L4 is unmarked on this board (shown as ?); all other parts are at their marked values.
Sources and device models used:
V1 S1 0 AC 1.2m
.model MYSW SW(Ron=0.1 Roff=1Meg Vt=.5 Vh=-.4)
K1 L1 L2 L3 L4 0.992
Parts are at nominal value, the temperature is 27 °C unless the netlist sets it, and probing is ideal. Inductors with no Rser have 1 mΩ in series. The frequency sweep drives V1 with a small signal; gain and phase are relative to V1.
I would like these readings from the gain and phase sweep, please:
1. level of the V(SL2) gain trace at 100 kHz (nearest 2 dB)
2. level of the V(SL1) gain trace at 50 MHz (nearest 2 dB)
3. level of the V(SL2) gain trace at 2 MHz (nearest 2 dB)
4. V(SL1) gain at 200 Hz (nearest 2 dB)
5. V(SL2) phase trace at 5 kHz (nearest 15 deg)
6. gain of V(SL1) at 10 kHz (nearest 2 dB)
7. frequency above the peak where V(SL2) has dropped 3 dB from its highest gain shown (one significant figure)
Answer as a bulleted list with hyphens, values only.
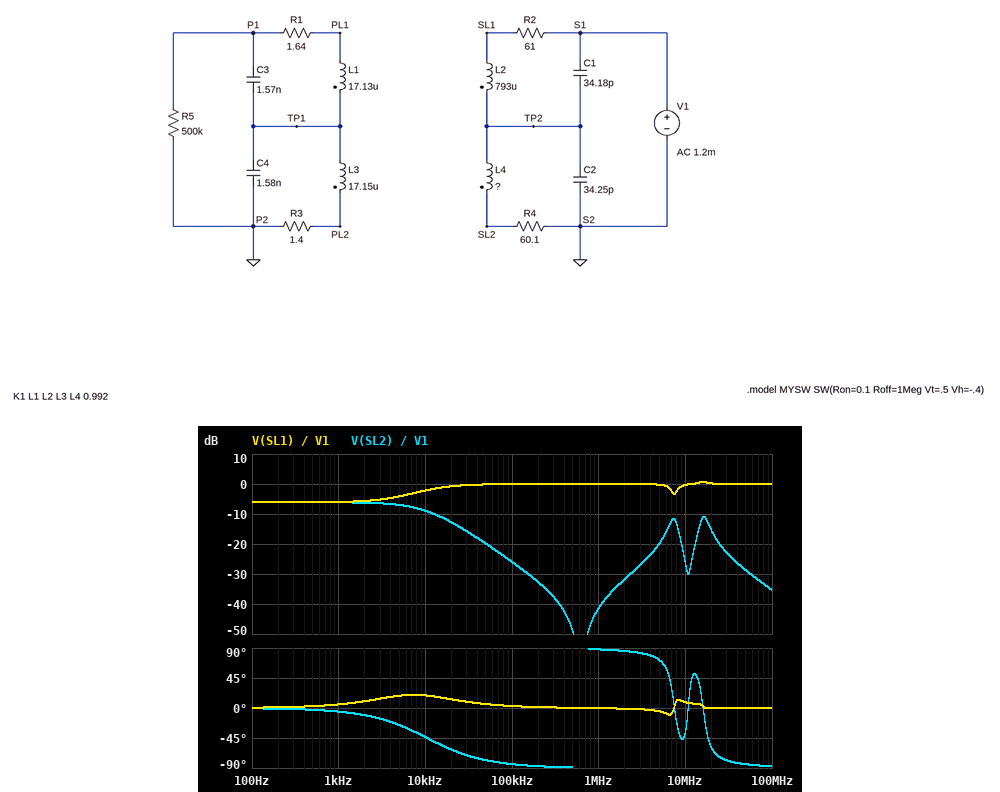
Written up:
- -26 dB
- 0 dB
- -32 dB
- -6 dB
- -30 deg
- -2 dB
- 10 kHz
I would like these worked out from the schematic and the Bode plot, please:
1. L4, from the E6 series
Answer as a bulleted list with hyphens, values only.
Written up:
- 220 µH
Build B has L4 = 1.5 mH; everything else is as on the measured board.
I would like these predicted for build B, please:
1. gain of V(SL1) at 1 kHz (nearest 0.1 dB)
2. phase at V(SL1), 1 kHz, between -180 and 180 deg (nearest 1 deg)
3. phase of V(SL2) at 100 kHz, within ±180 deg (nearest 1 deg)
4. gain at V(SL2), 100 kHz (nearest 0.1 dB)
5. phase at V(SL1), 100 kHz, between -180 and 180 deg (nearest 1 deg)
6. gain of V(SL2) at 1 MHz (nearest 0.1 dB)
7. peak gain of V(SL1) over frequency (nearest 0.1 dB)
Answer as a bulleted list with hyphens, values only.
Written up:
- -5.5 dB
- 12 deg
- -88 deg
- -33.5 dB
- 1 deg
- -56.0 dB
- 0 dB
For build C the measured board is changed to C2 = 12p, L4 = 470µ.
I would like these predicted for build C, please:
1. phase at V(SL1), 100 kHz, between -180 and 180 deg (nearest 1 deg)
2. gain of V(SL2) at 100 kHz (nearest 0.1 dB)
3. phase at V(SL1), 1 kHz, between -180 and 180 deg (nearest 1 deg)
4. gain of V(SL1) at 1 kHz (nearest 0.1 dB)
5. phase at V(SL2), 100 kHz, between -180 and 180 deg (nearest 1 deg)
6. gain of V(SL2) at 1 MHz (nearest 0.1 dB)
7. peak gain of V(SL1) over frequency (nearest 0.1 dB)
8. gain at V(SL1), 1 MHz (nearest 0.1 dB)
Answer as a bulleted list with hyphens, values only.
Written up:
- 2 deg
- -28.5 dB
- 7 deg
- -5.9 dB
- -86 deg
- -42.6 dB
- 2.0 dB
- 0 dB
